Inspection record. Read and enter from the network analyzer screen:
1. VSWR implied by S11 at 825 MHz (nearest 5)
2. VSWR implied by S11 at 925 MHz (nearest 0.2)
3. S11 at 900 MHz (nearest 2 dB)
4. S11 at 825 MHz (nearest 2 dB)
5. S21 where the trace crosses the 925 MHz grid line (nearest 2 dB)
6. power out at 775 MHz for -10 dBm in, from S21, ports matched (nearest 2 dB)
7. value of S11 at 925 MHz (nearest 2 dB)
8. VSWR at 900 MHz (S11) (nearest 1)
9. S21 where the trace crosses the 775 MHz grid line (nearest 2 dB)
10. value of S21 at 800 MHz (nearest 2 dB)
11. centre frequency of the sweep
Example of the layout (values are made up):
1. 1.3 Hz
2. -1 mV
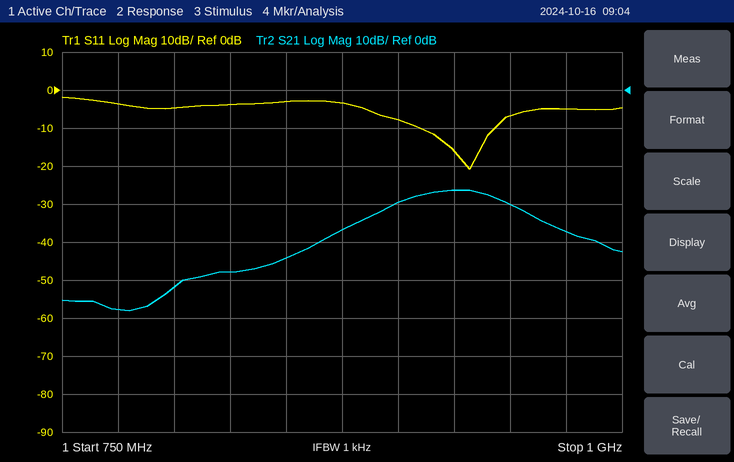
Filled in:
1. 5
2. 1.4
3. -8 dB
4. -4 dB
5. -26 dB
6. -68 dBm
7. -16 dB
8. 2
9. -58 dB
10. -52 dB
11. 875 MHz
